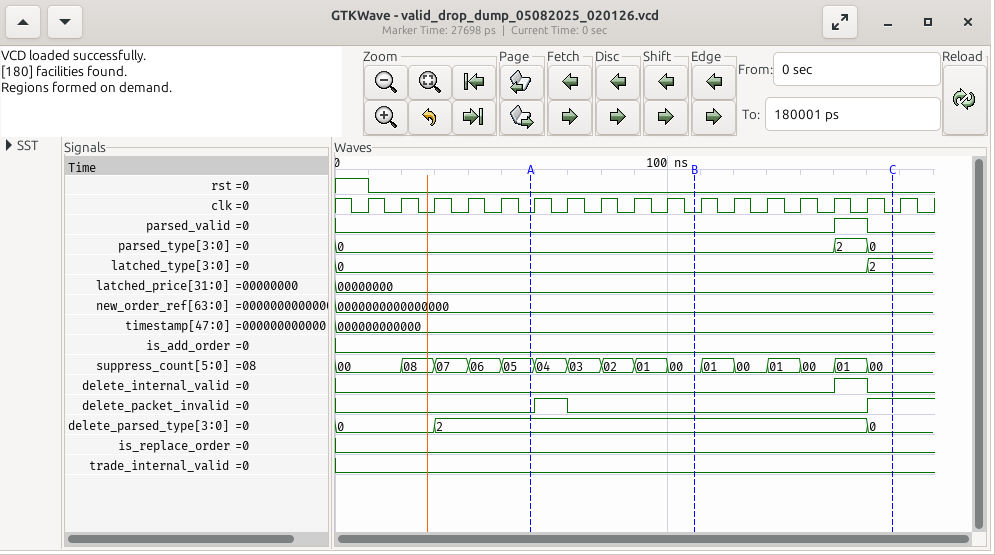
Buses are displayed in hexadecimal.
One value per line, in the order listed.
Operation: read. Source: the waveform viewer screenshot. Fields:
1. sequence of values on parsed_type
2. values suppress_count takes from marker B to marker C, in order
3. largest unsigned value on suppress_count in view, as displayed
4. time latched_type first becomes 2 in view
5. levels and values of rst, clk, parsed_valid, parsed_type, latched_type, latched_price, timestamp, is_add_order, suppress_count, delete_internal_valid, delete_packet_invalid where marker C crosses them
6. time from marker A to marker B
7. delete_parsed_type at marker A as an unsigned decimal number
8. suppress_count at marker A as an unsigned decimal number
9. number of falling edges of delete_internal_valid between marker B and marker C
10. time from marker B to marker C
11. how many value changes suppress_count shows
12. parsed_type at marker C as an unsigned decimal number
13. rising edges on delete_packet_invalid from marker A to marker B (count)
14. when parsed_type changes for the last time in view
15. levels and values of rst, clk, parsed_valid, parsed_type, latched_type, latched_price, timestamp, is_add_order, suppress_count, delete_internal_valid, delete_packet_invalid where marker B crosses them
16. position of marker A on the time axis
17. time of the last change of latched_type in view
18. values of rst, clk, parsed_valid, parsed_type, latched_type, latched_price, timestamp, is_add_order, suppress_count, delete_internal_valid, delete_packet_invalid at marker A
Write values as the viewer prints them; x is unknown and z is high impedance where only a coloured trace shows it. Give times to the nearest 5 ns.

0, 2, 0
00, 01, 00, 01, 00, 01, 00
08
160 ns
rst=0, clk=0, parsed_valid=0, parsed_type=0, latched_type=2, latched_price=00000000, timestamp=000000000000, is_add_order=0, suppress_count=00, delete_internal_valid=0, delete_packet_invalid=1
50 ns
2
5
1
60 ns
15
0
1
160 ns
rst=0, clk=0, parsed_valid=0, parsed_type=0, latched_type=0, latched_price=00000000, timestamp=000000000000, is_add_order=0, suppress_count=00, delete_internal_valid=0, delete_packet_invalid=0
60 ns
160 ns
rst=0, clk=0, parsed_valid=0, parsed_type=0, latched_type=0, latched_price=00000000, timestamp=000000000000, is_add_order=0, suppress_count=05, delete_internal_valid=0, delete_packet_invalid=0
